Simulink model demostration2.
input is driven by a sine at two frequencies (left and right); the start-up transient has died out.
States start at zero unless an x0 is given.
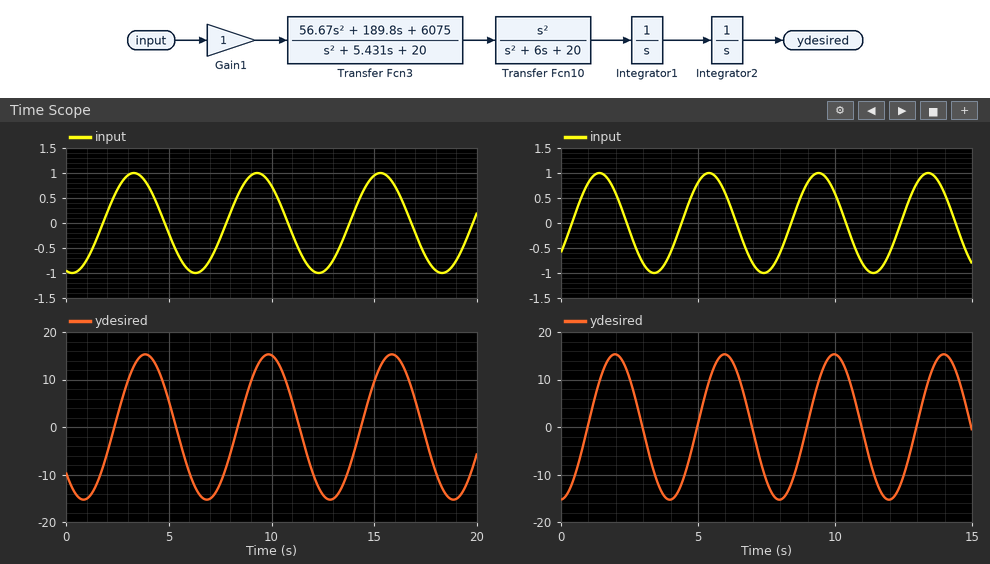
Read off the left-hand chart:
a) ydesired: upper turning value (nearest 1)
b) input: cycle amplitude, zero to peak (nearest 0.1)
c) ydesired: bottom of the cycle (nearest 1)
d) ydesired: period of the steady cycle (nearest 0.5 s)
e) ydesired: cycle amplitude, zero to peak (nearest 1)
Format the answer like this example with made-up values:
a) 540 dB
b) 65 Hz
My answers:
a) 15
b) 1.0
c) -15
d) 6.0 s
e) 15
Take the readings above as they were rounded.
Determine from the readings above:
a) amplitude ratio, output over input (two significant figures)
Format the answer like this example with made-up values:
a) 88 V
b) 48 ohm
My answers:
a) 15
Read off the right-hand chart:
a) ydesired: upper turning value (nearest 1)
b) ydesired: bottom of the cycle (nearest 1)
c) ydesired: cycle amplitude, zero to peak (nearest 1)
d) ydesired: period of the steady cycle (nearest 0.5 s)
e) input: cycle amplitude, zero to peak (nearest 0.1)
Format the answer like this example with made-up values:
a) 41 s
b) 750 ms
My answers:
a) 15
b) -15
c) 15
d) 4.0 s
e) 1.0
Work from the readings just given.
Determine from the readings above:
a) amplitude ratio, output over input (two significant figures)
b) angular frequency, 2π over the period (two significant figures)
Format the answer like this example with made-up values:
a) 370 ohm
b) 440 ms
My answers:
a) 15
b) 1.6 rad/s
